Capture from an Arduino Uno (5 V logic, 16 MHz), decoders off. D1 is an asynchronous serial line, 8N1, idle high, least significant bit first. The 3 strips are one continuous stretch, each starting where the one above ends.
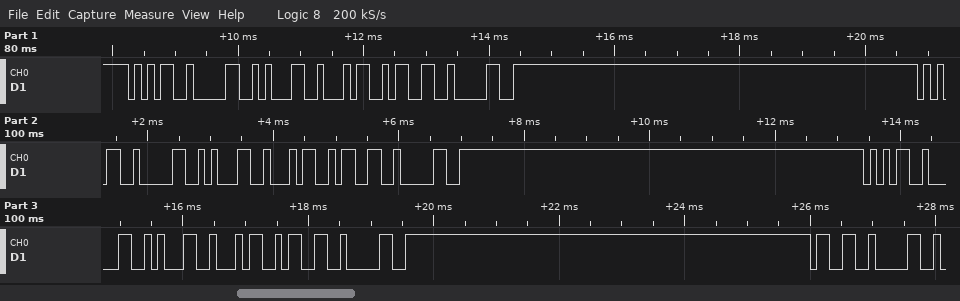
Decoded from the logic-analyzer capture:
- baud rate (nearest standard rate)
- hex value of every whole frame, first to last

9600 baud
35 30 31 34 33 30 35 30 31 34 33 30 35 30 31 34 33 30 33 30
